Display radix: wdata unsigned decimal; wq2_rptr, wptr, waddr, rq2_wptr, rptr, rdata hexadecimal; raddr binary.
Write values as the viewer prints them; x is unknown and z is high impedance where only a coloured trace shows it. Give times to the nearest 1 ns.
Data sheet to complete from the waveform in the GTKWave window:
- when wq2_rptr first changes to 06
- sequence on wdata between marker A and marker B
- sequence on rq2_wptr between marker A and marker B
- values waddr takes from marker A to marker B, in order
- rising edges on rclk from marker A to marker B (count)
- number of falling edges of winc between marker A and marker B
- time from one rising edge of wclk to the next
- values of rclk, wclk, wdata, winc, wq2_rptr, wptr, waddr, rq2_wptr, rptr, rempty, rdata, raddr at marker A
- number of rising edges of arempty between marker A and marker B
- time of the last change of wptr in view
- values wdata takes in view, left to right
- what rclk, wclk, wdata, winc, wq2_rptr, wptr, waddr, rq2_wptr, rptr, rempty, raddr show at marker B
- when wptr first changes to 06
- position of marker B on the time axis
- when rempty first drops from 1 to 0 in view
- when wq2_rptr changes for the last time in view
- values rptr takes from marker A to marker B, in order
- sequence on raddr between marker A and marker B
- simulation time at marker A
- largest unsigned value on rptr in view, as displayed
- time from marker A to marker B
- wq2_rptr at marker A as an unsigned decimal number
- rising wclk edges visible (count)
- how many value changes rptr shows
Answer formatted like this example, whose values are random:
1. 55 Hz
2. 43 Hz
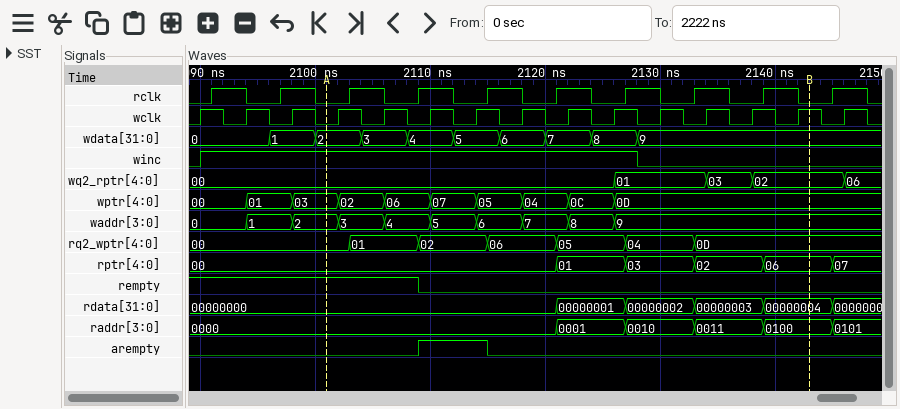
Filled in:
1. 2146 ns
2. 2, 3, 4, 5, 6, 7, 8, 9
3. 00, 01, 02, 06, 05, 04, 0D
4. 2, 3, 4, 5, 6, 7, 8, 9
5. 7
6. 1
7. 4 ns
8. rclk=0, wclk=0, wdata=2, winc=1, wq2_rptr=00, wptr=03, waddr=2, rq2_wptr=00, rptr=00, rempty=1, rdata=00000000, raddr=0000
9. 1
10. 2126 ns
11. 0, 1, 2, 3, 4, 5, 6, 7, 8, 9
12. rclk=0, wclk=1, wdata=9, winc=0, wq2_rptr=02, wptr=0D, waddr=9, rq2_wptr=0D, rptr=06, rempty=0, raddr=0100
13. 2106 ns
14. 2143 ns
15. 2109 ns
16. 2146 ns
17. 00, 01, 03, 02, 06
18. 0000, 0001, 0010, 0011, 0100
19. 2101 ns
20. 07
21. 42 ns
22. 0
23. 15
24. 5
